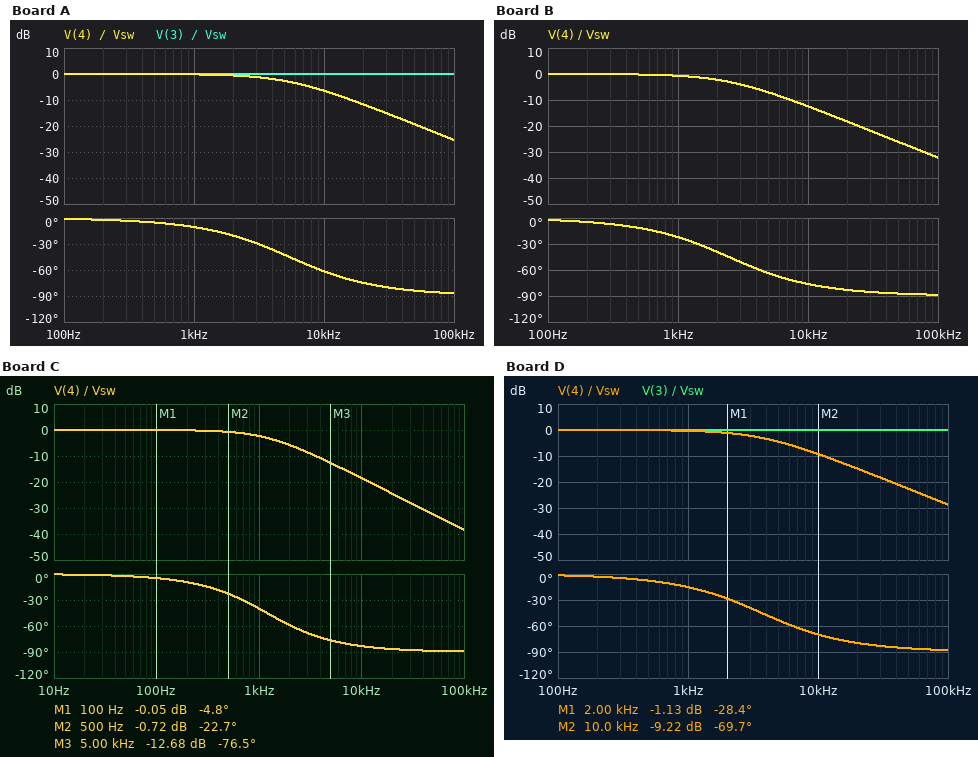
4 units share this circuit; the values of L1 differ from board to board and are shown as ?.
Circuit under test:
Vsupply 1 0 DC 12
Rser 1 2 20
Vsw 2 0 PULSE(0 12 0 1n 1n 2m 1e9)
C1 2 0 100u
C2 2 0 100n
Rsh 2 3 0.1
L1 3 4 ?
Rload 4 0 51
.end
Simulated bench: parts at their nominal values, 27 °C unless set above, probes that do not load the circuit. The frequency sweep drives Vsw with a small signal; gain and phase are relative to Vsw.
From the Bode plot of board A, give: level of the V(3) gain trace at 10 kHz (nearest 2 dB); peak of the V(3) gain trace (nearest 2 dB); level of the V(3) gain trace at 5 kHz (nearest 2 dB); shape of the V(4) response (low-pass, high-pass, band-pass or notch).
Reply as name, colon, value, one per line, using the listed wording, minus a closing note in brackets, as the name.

level of the V(3) gain trace at 10 kHz: 0 dB
peak of the V(3) gain trace: 0 dB
level of the V(3) gain trace at 5 kHz: 0 dB
shape of the V(4) response: low-pass
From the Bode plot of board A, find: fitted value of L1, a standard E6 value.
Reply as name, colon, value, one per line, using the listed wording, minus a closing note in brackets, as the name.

fitted value of L1, a standard E6 value: 1.5 mH
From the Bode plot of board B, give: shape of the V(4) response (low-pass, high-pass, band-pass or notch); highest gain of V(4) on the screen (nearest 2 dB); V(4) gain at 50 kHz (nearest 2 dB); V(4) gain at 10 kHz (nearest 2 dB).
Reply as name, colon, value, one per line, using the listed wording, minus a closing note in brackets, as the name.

shape of the V(4) response: low-pass
highest gain of V(4) on the screen: 0 dB
V(4) gain at 50 kHz: -26 dB
V(4) gain at 10 kHz: -12 dB
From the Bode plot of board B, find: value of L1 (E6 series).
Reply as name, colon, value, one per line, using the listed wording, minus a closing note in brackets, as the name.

value of L1: 3.3 mH
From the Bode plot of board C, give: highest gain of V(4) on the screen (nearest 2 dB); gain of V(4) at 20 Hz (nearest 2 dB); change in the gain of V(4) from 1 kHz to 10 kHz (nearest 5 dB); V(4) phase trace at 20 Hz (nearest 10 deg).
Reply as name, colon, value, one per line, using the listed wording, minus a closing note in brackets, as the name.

highest gain of V(4) on the screen: 0 dB
gain of V(4) at 20 Hz: 0 dB
change in the gain of V(4) from 1 kHz to 10 kHz: -15 dB
V(4) phase trace at 20 Hz: 0 deg
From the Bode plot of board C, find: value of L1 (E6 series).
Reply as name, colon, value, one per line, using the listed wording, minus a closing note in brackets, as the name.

value of L1: 6.8 mH
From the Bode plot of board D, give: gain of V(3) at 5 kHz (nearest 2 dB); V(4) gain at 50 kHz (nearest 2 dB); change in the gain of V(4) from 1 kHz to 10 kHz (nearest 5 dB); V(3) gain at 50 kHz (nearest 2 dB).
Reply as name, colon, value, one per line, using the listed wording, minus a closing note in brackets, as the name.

gain of V(3) at 5 kHz: 0 dB
V(4) gain at 50 kHz: -22 dB
change in the gain of V(4) from 1 kHz to 10 kHz: -10 dB
V(3) gain at 50 kHz: 0 dB
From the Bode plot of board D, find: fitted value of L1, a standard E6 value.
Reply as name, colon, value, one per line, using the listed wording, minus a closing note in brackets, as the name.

fitted value of L1, a standard E6 value: 2.2 mH
